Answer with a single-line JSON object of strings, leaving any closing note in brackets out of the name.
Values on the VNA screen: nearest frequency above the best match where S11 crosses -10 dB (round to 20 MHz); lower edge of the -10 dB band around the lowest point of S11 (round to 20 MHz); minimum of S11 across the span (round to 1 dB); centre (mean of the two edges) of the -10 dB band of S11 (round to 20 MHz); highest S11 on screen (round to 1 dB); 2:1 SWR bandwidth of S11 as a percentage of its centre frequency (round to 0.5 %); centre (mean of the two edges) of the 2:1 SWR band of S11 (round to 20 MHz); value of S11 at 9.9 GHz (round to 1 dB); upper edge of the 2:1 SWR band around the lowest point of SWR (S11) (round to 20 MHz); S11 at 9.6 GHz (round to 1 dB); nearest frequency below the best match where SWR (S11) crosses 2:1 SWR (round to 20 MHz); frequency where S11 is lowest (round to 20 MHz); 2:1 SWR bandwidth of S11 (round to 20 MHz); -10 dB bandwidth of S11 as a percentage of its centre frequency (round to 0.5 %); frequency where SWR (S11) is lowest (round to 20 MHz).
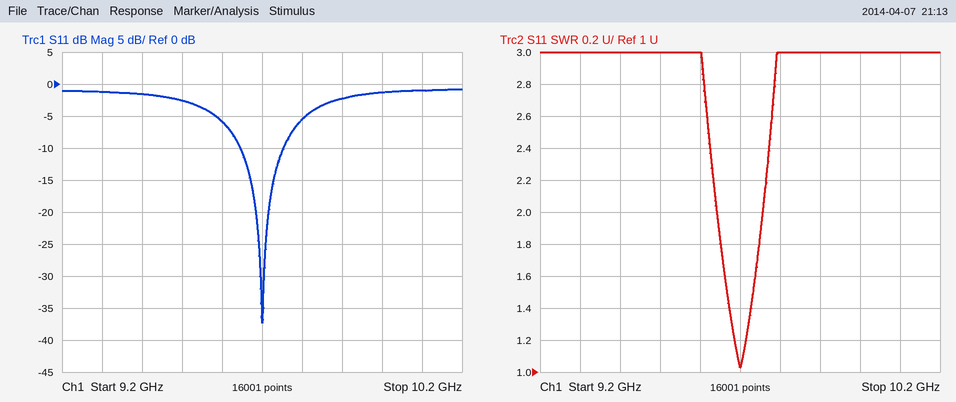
{"nearest frequency above the best match where S11 crosses -10 dB": "9.76 GHz", "lower edge of the -10 dB band around the lowest point of S11": "9.64 GHz", "minimum of S11 across the span": "-37 dB", "centre (mean of the two edges) of the -10 dB band of S11": "9.70 GHz", "highest S11 on screen": "-1 dB", "2:1 SWR bandwidth of S11 as a percentage of its centre frequency": "1.0 %", "centre (mean of the two edges) of the 2:1 SWR band of S11": "9.70 GHz", "value of S11 at 9.9 GHz": "-2 dB", "upper edge of the 2:1 SWR band around the lowest point of SWR (S11)": "9.76 GHz", "S11 at 9.6 GHz": "-6 dB", "nearest frequency below the best match where SWR (S11) crosses 2:1 SWR": "9.64 GHz", "frequency where S11 is lowest": "9.70 GHz", "2:1 SWR bandwidth of S11": "120 MHz", "-10 dB bandwidth of S11 as a percentage of its centre frequency": "1.0 %", "frequency where SWR (S11) is lowest": "9.70 GHz"}
